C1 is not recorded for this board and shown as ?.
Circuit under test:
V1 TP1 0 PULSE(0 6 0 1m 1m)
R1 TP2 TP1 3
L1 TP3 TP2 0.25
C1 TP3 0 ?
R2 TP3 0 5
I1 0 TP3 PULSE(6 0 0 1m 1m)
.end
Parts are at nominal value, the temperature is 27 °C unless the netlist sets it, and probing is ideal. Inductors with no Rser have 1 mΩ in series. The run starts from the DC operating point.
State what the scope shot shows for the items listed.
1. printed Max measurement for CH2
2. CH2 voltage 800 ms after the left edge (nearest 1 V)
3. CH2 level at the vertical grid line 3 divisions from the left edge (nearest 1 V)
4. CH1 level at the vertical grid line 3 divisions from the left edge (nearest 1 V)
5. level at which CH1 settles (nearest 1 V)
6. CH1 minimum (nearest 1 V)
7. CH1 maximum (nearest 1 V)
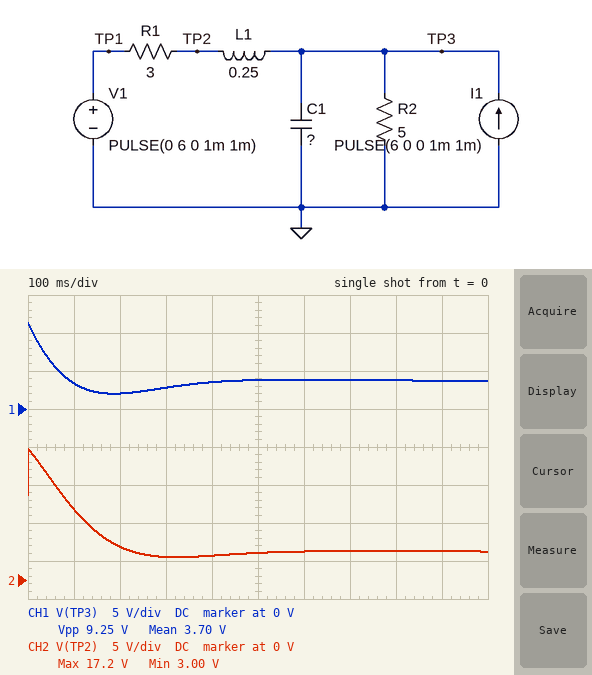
17.2 V
4 V
3 V
3 V
4 V
2 V
11 V
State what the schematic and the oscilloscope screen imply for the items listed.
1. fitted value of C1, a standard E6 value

47 mF
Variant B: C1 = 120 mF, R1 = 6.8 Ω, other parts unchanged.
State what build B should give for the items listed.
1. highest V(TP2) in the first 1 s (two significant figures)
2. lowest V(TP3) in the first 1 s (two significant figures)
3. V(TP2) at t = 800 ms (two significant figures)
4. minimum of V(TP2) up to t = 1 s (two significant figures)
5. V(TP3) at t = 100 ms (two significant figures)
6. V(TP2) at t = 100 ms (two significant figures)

23 V
3.2 V
4.0 V
3.3 V
13 V
15 V
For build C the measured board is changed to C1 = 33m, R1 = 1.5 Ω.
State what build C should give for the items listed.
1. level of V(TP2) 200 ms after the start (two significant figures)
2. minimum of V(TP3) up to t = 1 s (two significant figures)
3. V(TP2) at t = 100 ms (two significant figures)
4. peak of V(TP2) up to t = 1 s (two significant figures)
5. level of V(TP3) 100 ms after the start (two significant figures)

3.5 V
-2.3 V
7.3 V
13 V
-2.2 V
